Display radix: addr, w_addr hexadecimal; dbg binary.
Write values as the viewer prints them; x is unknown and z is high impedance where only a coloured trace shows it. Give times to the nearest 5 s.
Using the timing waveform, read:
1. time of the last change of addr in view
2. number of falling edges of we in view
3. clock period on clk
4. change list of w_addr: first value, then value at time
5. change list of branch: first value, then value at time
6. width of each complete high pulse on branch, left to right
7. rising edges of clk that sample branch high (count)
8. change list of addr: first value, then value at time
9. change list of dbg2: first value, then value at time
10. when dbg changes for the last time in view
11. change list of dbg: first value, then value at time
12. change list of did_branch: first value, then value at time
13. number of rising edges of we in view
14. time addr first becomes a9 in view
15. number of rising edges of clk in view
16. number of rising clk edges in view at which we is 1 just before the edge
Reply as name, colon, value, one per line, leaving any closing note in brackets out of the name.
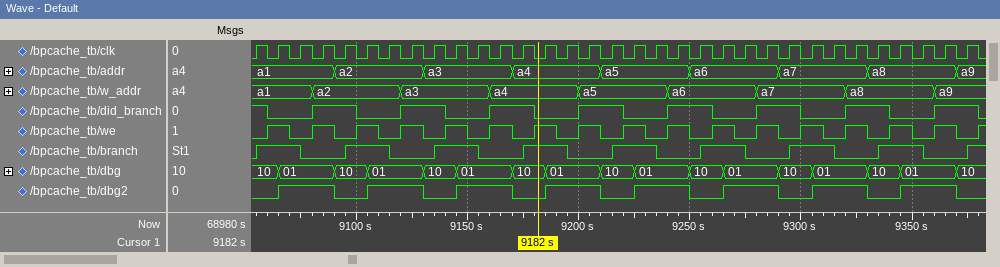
time of the last change of addr in view: 9370 s
number of falling edges of we in view: 16
clock period on clk: 10 s
change list of w_addr: first value, then value at time: a1, a2 at 9080 s, a3 at 9120 s, a4 at 9160 s, a5 at 9200 s, a6 at 9240 s, a7 at 9280 s, a8 at 9320 s, a9 at 9360 s
change list of branch: first value, then value at time: 0, 1 at 9055 s, 0 at 9075 s, 1 at 9095 s, 0 at 9115 s, 1 at 9135 s, 0 at 9155 s, 1 at 9175 s, 0 at 9195 s, 1 at 9215 s, 0 at 9235 s, 1 at 9255 s, 0 at 9275 s, 1 at 9295 s, 0 at 9315 s, 1 at 9335 s, 0 at 9355 s, 1 at 9375 s
width of each complete high pulse on branch, left to right: 20 s, 20 s, 20 s, 20 s, 20 s, 20 s, 20 s, 20 s
rising edges of clk that sample branch high: 16
change list of addr: first value, then value at time: a1, a2 at 9090 s, a3 at 9130 s, a4 at 9170 s, a5 at 9210 s, a6 at 9250 s, a7 at 9290 s, a8 at 9330 s, a9 at 9370 s
change list of dbg2: first value, then value at time: 0, 1 at 9065 s, 0 at 9090 s, 1 at 9105 s, 0 at 9130 s, 1 at 9145 s, 0 at 9170 s, 1 at 9185 s, 0 at 9210 s, 1 at 9225 s, 0 at 9250 s, 1 at 9265 s, 0 at 9290 s, 1 at 9305 s, 0 at 9330 s, 1 at 9345 s, 0 at 9370 s
when dbg changes for the last time in view: 9370 s
change list of dbg: first value, then value at time: 10, 01 at 9065 s, 10 at 9090 s, 01 at 9105 s, 10 at 9130 s, 01 at 9145 s, 10 at 9170 s, 01 at 9185 s, 10 at 9210 s, 01 at 9225 s, 10 at 9250 s, 01 at 9265 s, 10 at 9290 s, 01 at 9305 s, 10 at 9330 s, 01 at 9345 s, 10 at 9370 s
change list of did_branch: first value, then value at time: 1, 0 at 9060 s, 1 at 9080 s, 0 at 9100 s, 1 at 9120 s, 0 at 9140 s, 1 at 9160 s, 0 at 9180 s, 1 at 9200 s, 0 at 9220 s, 1 at 9240 s, 0 at 9260 s, 1 at 9280 s, 0 at 9300 s, 1 at 9320 s, 0 at 9340 s, 1 at 9360 s, 0 at 9380 s
number of rising edges of we in view: 17
time addr first becomes a9 in view: 9370 s
number of rising edges of clk in view: 33
number of rising clk edges in view at which we is 1 just before the edge: 16
